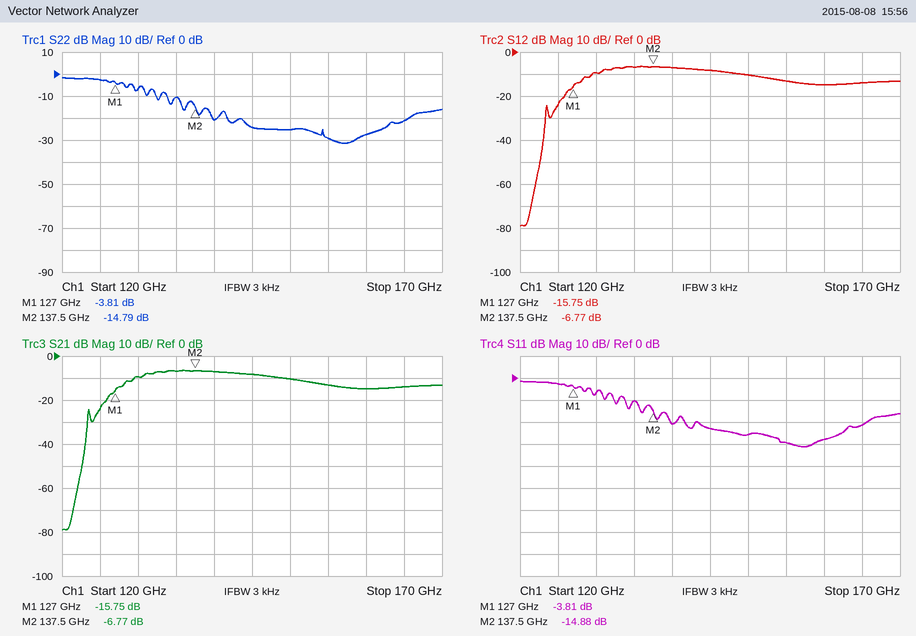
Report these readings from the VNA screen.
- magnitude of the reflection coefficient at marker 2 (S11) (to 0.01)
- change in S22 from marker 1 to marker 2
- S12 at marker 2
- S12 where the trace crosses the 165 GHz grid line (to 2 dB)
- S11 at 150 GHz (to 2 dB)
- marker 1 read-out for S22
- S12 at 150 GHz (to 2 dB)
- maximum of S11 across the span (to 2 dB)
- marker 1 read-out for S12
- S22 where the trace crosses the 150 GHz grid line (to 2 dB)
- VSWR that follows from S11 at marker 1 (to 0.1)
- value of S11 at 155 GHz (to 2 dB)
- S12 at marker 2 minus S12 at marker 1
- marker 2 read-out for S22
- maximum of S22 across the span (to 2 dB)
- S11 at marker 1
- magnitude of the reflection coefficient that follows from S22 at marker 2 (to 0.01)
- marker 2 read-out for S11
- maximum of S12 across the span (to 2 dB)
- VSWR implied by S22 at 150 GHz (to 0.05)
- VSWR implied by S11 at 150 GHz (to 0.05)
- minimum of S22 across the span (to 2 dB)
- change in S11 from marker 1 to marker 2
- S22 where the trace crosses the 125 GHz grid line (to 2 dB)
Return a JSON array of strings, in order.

["0.18", "-10.98 dB", "-6.77 dB", "-14 dB", "-26 dB", "-3.81 dB", "-10 dB", "-2 dB", "-15.75 dB", "-26 dB", "4.6", "-30 dB", "8.98 dB", "-14.79 dB", "-2 dB", "-3.81 dB", "0.18", "-14.88 dB", "-6 dB", "1.10", "1.10", "-32 dB", "-11.07 dB", "-2 dB"]
